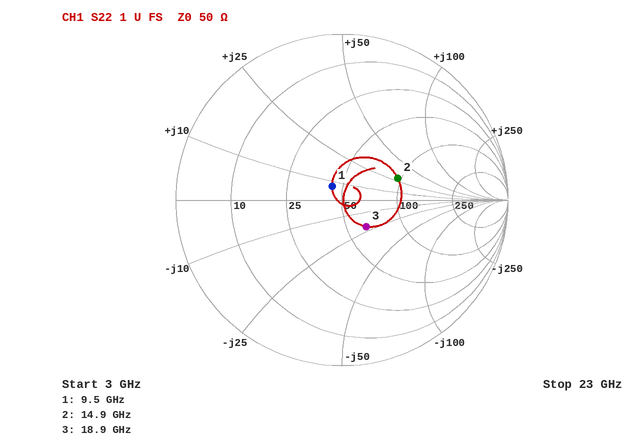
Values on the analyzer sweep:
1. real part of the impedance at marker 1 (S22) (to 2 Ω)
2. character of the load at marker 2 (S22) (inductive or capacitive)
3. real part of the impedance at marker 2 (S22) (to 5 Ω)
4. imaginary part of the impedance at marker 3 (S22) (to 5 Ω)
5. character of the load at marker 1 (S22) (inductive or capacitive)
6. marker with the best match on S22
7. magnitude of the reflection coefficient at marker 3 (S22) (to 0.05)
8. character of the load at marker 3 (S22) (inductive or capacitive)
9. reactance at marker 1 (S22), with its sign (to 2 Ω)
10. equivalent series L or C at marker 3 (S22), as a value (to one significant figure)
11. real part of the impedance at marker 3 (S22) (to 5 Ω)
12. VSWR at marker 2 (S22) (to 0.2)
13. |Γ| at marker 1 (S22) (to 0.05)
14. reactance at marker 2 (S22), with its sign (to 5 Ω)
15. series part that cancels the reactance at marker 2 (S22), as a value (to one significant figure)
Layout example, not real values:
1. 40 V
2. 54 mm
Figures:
1. 44 Ω
2. inductive
3. 95 Ω
4. -20 Ω
5. inductive
6. marker 1
7. 0.20
8. capacitive
9. +8 Ω
10. 400 fF
11. 65 Ω
12. 2.2
13. 0.10
14. +30 Ω
15. 400 fF
